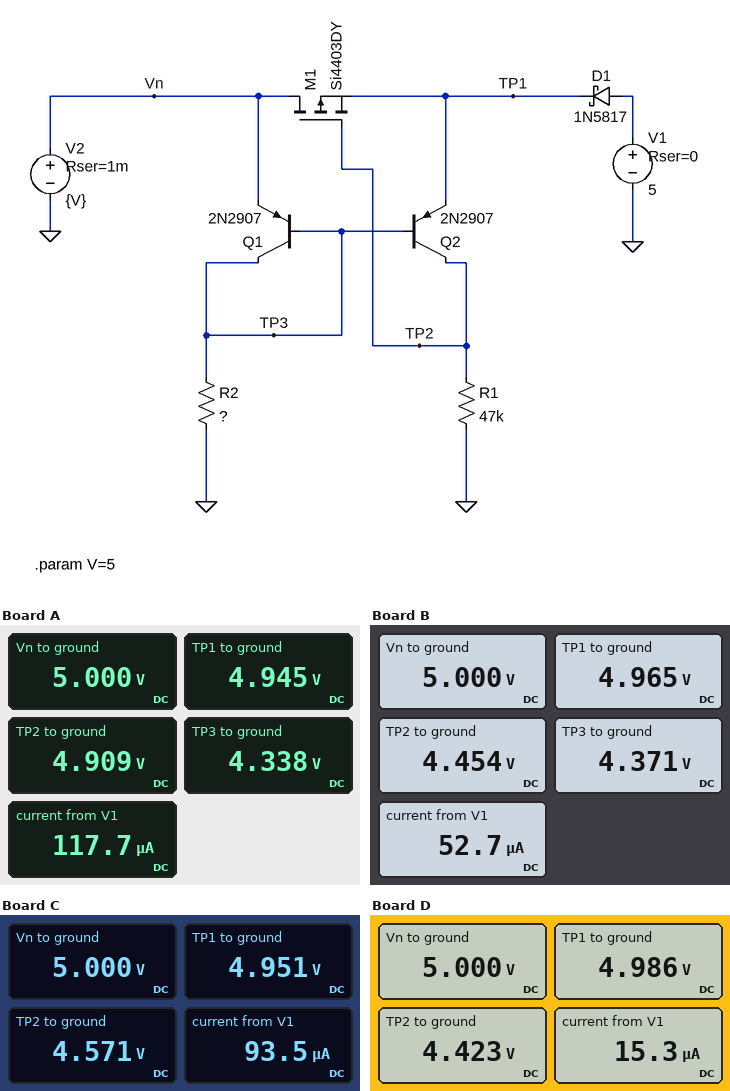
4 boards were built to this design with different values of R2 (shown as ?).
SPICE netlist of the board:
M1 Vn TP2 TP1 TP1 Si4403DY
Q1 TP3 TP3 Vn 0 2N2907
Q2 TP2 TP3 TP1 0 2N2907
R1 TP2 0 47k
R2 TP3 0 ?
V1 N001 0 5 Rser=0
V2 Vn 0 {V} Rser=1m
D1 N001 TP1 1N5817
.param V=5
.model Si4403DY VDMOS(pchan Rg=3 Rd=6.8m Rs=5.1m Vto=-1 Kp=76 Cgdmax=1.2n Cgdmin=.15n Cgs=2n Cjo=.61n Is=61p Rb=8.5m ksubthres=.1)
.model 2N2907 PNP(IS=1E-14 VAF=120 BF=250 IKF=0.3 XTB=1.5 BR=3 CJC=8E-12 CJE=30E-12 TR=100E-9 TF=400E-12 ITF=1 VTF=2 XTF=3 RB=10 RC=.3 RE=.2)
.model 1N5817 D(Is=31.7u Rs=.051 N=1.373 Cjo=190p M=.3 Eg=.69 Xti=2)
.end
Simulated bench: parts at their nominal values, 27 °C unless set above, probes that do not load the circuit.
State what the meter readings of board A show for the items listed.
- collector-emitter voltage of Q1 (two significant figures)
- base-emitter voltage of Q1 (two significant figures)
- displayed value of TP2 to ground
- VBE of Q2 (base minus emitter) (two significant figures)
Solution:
-660 mV
-660 mV
4.909 V
-610 mV
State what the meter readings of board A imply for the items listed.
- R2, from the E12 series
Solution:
3.3 kΩ
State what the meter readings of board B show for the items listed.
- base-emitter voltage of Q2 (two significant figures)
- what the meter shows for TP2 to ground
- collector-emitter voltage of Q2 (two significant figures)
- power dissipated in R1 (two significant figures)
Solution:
-590 mV
4.454 V
-510 mV
420 µW
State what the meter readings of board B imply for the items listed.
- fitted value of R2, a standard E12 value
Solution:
12 kΩ
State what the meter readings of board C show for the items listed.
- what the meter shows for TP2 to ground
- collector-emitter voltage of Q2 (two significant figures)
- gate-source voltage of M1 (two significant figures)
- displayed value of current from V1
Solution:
4.571 V
-380 mV
-380 mV
93.5 µA
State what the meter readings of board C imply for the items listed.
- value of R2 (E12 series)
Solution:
6.8 kΩ
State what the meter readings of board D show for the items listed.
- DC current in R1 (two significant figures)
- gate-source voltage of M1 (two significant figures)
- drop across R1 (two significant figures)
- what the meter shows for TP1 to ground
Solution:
94 µA
-560 mV
4.4 V
4.986 V
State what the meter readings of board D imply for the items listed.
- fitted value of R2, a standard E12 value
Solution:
27 kΩ
